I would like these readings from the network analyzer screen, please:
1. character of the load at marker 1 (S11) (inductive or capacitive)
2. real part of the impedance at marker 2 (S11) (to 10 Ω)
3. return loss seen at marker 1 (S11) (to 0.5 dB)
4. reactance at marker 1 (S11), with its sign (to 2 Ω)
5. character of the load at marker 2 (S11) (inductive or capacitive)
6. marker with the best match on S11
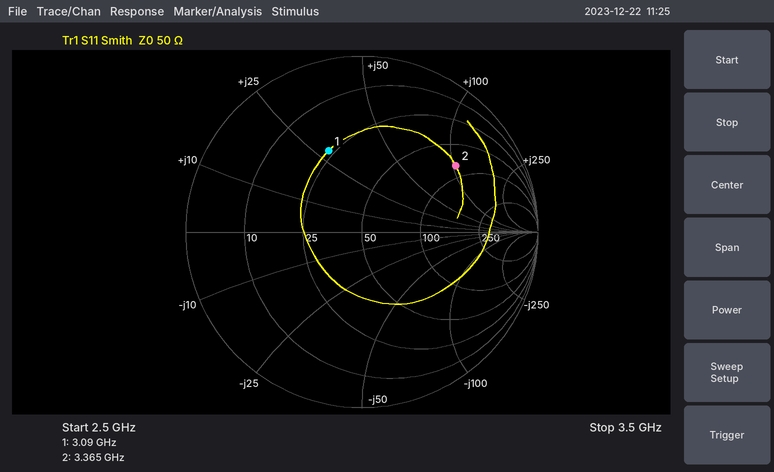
inductive
80 Ω
6.0 dB
+28 Ω
inductive
marker 1
